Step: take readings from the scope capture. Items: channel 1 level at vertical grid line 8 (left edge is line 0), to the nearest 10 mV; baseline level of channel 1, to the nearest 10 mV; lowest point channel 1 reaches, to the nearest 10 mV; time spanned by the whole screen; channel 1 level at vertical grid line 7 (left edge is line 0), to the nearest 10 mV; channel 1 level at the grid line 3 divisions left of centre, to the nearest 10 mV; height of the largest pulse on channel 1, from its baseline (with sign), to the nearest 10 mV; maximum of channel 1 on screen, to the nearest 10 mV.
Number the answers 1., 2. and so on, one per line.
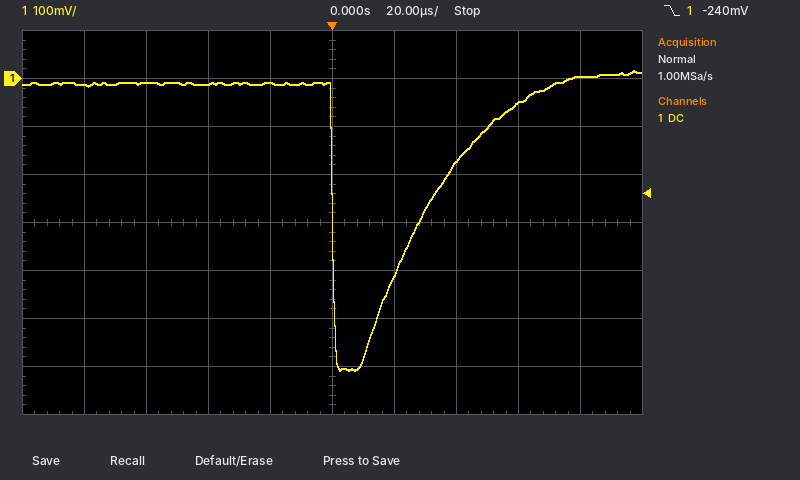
1. -50 mV
2. -10 mV
3. -610 mV
4. 200 µs
5. -170 mV
6. -10 mV
7. -600 mV
8. 20 mV
